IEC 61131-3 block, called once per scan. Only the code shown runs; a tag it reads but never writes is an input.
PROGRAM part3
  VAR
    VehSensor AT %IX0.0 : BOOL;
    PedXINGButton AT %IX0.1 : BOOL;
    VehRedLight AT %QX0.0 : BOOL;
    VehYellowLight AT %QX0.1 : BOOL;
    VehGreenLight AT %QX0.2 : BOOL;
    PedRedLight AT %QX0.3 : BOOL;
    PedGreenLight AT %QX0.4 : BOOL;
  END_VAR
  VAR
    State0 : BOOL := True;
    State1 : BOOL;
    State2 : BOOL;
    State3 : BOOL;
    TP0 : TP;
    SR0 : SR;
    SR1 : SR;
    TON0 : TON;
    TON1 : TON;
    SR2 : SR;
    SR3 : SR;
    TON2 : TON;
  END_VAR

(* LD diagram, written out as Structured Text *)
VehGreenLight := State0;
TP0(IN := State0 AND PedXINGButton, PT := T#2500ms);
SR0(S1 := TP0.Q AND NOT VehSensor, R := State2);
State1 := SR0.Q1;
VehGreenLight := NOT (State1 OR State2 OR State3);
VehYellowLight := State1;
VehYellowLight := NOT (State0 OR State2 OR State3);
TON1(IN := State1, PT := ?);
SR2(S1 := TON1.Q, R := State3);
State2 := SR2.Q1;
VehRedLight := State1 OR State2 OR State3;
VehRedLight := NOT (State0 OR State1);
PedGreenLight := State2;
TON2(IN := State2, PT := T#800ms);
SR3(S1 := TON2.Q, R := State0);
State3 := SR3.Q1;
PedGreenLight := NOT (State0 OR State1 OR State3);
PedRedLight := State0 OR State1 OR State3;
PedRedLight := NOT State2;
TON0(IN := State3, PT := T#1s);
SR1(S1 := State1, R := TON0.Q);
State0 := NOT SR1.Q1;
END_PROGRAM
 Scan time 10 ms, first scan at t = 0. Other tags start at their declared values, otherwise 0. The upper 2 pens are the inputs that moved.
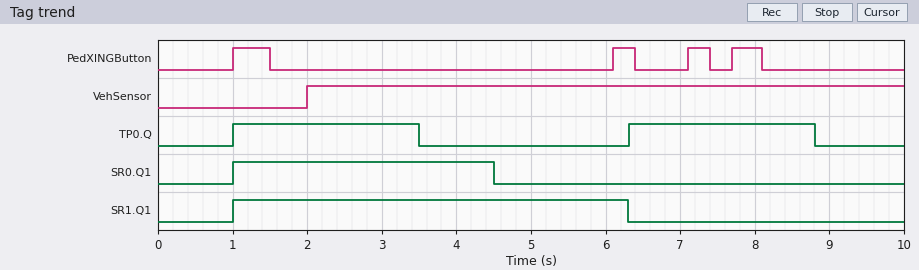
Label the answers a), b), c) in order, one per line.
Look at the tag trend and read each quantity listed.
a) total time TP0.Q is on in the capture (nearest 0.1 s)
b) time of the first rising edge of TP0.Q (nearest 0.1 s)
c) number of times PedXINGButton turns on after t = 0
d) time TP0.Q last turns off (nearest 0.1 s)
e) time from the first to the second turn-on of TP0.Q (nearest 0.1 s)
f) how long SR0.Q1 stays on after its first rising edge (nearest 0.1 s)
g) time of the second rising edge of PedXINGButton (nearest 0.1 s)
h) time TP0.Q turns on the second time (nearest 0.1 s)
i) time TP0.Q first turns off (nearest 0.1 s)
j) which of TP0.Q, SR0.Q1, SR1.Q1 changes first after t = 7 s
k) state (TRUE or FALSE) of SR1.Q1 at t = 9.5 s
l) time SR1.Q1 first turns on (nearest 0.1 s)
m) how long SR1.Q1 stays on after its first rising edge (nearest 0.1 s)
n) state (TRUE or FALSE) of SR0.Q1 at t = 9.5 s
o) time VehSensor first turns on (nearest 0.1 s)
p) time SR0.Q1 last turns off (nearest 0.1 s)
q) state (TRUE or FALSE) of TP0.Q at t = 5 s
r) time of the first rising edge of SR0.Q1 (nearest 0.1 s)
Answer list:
a) 5.0 s
b) 1.0 s
c) 4
d) 8.8 s
e) 5.3 s
f) 3.5 s
g) 6.1 s
h) 6.3 s
i) 3.5 s
j) TP0.Q
k) FALSE
l) 1.0 s
m) 5.3 s
n) FALSE
o) 2.0 s
p) 4.5 s
q) FALSE
r) 1.0 s
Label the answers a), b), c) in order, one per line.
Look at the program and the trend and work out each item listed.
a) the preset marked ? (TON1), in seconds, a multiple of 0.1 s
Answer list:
a) 3.5 s
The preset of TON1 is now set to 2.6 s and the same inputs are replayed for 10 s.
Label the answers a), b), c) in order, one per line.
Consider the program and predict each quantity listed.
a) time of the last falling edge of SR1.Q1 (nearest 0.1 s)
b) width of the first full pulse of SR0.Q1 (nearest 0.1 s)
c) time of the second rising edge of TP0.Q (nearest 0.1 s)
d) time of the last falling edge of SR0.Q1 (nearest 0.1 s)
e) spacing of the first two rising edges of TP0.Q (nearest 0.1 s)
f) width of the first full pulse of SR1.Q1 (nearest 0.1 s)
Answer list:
a) 5.4 s
b) 2.6 s
c) 6.1 s
d) 3.6 s
e) 5.1 s
f) 4.4 s
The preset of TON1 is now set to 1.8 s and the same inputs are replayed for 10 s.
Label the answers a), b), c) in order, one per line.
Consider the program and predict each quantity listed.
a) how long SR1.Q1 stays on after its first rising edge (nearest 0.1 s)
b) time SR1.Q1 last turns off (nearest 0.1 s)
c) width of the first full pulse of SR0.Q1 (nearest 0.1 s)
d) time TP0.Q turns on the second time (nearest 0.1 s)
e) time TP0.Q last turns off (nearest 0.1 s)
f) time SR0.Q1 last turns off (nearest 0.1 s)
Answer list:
a) 3.6 s
b) 4.6 s
c) 1.8 s
d) 6.1 s
e) 8.6 s
f) 2.8 s
